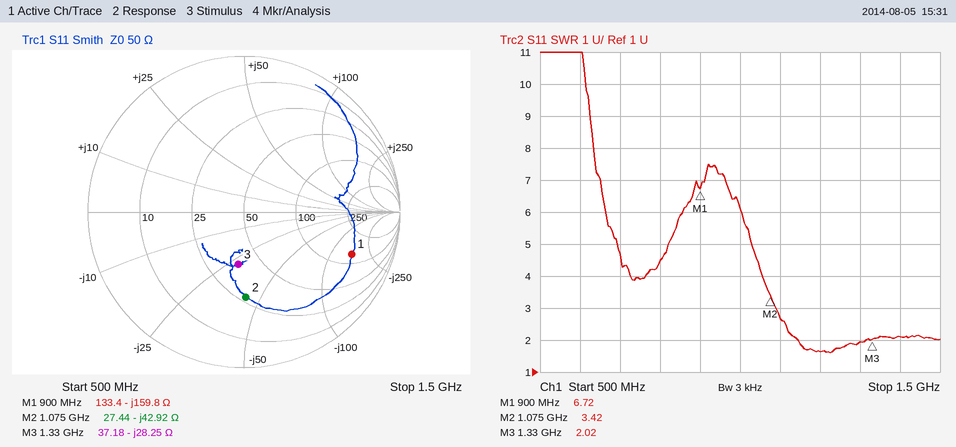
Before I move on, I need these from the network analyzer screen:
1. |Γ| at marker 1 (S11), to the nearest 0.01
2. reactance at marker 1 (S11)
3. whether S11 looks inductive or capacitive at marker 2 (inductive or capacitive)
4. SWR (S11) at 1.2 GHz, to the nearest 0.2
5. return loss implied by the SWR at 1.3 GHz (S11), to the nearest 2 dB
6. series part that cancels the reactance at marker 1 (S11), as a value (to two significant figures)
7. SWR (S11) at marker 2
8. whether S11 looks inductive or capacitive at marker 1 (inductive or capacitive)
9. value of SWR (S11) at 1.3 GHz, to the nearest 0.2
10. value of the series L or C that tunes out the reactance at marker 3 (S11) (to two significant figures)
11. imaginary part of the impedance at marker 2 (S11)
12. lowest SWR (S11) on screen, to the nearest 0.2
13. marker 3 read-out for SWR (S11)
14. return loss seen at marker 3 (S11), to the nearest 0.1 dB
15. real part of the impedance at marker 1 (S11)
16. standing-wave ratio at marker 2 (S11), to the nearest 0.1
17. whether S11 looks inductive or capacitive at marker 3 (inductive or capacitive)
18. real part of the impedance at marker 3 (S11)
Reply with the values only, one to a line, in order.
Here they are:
0.74
-159.8 Ω
capacitive
1.6
10 dB
28 nH
3.42
capacitive
2.0
3.4 nH
-42.92 Ω
1.6
2.02
9.4 dB
133.4 Ω
3.4
capacitive
37.18 Ω
